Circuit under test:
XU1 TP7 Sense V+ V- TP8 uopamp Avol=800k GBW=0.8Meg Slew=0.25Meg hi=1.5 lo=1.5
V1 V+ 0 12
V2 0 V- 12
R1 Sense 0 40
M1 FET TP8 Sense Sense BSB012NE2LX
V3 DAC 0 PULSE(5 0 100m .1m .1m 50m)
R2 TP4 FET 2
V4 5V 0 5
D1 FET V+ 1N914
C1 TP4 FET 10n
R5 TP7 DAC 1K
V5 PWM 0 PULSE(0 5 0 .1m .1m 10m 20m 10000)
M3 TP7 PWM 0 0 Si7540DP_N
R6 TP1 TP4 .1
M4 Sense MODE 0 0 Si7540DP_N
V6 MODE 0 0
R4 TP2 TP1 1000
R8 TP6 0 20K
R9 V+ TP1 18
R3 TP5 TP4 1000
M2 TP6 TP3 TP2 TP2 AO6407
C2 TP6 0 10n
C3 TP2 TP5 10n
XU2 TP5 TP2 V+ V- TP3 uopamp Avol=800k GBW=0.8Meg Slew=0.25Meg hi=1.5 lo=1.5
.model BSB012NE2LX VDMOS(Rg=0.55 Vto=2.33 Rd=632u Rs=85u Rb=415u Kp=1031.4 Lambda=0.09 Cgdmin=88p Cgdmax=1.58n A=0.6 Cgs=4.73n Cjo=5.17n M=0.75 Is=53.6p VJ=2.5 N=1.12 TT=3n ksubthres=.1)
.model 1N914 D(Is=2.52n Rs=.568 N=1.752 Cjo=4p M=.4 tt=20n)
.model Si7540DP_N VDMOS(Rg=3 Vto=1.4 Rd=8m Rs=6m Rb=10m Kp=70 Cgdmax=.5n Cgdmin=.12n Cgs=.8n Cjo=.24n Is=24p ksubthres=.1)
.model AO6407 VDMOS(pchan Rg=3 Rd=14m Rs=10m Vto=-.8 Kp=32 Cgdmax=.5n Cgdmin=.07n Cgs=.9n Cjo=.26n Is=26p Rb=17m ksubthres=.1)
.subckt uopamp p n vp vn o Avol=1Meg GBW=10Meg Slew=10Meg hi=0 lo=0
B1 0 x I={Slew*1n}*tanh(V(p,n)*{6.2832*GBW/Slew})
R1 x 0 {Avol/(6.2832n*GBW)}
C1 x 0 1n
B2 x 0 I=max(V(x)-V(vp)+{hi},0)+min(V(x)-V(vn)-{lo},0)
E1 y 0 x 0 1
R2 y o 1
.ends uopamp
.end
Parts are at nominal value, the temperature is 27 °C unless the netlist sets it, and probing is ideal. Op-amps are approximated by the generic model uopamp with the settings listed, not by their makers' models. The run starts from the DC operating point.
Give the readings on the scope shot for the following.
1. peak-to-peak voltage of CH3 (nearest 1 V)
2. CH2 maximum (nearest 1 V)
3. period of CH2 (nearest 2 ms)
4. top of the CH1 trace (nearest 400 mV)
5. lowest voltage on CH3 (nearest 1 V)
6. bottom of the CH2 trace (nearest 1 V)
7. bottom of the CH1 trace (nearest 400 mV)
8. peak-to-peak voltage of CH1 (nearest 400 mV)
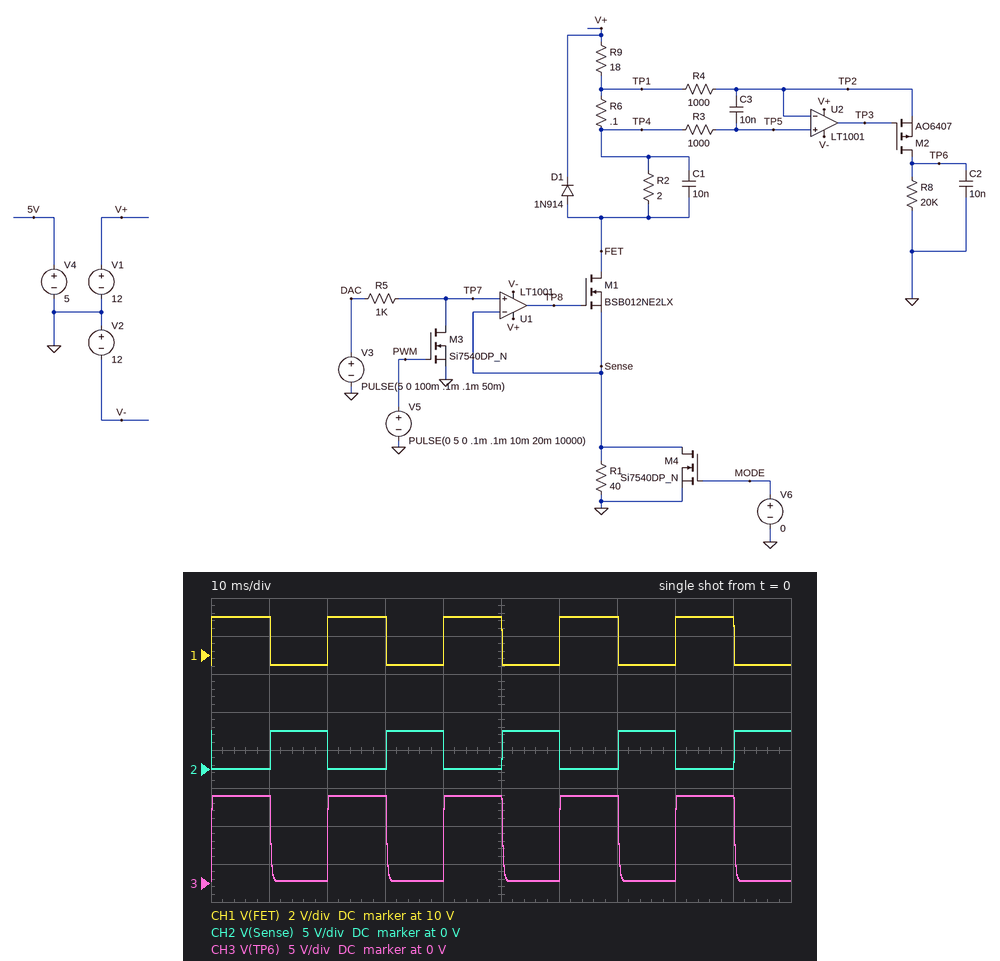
11 V
5 V
20 ms
12.0 V
0 V
0 V
9.6 V
2.4 V
